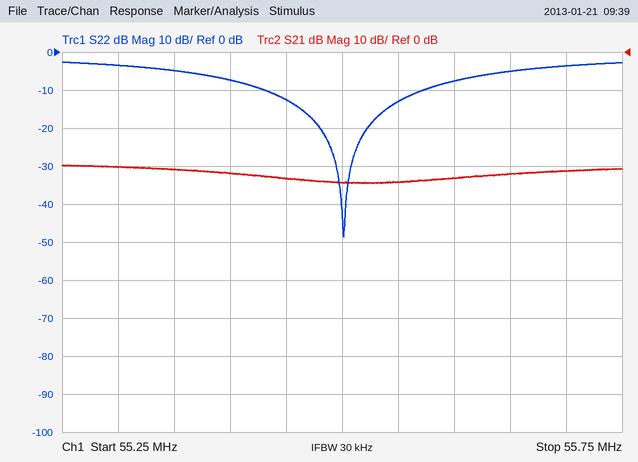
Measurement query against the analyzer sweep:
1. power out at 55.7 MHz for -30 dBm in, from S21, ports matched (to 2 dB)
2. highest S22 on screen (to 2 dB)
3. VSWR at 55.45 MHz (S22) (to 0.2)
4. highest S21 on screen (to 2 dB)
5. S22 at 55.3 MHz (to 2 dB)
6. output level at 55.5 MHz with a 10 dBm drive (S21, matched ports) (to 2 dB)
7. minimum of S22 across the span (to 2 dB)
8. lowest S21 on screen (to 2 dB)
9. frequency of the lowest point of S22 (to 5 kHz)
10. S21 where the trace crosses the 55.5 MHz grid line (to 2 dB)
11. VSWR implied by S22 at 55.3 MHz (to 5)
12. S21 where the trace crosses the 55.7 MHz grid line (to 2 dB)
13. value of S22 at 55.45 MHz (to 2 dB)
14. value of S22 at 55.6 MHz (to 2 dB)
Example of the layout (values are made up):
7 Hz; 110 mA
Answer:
-62 dBm; -2 dB; 1.6; -30 dB; -4 dB; -24 dBm; -48 dB; -34 dB; 55.500 MHz; -34 dB; 5; -32 dB; -12 dB; -8 dB
